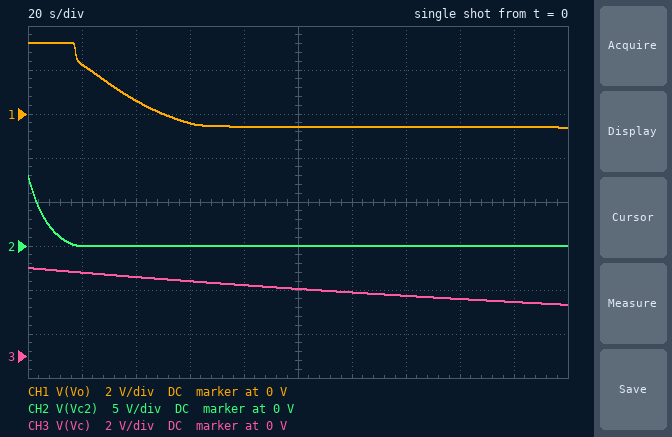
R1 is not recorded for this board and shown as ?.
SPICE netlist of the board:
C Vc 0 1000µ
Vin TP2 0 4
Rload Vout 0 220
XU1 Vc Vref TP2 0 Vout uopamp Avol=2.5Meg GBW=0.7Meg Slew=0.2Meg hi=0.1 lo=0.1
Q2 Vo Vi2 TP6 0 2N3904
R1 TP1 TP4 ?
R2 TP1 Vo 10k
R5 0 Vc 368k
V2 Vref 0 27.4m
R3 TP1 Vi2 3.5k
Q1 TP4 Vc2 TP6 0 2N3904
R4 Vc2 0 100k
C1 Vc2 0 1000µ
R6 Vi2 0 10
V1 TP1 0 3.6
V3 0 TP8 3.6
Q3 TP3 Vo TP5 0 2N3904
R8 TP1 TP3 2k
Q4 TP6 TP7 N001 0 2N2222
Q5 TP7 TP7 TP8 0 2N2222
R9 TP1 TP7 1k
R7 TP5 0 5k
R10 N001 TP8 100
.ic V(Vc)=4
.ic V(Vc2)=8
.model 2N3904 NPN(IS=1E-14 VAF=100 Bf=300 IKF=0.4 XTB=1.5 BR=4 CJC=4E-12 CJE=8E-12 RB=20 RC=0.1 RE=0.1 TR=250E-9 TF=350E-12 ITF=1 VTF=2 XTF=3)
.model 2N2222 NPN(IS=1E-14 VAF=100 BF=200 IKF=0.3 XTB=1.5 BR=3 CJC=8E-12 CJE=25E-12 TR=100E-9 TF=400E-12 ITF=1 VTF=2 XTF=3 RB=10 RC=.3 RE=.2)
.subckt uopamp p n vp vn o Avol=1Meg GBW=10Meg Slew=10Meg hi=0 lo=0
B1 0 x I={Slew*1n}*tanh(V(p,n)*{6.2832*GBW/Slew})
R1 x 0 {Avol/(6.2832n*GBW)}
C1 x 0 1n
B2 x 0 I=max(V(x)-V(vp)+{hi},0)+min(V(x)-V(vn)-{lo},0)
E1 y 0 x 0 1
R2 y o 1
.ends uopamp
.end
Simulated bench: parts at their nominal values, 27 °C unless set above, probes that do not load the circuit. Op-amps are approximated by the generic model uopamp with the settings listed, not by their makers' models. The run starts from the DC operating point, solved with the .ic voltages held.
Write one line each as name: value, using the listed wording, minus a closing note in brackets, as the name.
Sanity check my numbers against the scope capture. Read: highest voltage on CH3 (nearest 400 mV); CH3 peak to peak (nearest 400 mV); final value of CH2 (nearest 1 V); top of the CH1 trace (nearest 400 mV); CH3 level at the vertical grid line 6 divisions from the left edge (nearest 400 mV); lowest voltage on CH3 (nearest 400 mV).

highest voltage on CH3: 4.0 V
CH3 peak to peak: 1.6 V
final value of CH2: 0 V
top of the CH1 trace: 3.2 V
CH3 level at the vertical grid line 6 divisions from the left edge: 2.8 V
lowest voltage on CH3: 2.4 V
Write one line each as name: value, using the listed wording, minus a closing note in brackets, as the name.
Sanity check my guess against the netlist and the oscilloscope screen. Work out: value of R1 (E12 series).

value of R1: 8.2 kΩ
